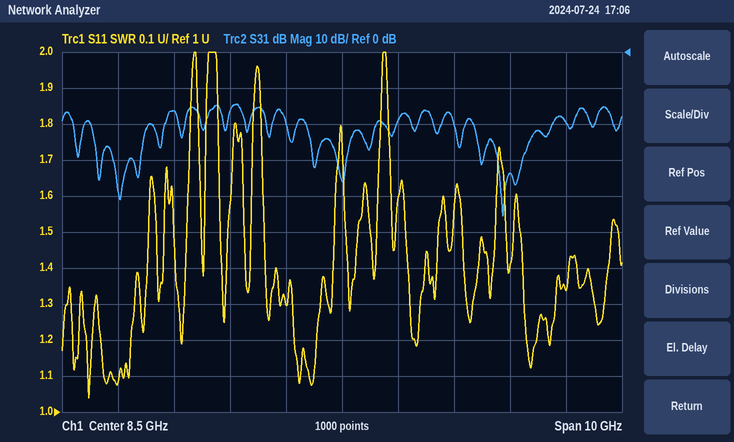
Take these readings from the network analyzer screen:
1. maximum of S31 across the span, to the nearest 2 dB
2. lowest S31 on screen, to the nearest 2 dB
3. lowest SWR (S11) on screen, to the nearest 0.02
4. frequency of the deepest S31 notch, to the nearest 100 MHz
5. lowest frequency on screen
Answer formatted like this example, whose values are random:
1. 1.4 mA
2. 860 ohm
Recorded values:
1. -14 dB
2. -46 dB
3. 1.04
4. 11.4 GHz
5. 3.5 GHz
